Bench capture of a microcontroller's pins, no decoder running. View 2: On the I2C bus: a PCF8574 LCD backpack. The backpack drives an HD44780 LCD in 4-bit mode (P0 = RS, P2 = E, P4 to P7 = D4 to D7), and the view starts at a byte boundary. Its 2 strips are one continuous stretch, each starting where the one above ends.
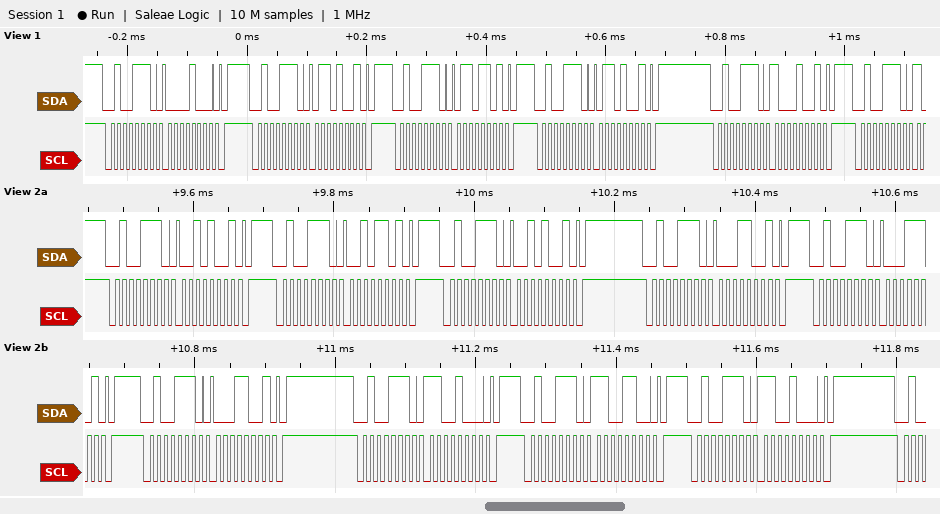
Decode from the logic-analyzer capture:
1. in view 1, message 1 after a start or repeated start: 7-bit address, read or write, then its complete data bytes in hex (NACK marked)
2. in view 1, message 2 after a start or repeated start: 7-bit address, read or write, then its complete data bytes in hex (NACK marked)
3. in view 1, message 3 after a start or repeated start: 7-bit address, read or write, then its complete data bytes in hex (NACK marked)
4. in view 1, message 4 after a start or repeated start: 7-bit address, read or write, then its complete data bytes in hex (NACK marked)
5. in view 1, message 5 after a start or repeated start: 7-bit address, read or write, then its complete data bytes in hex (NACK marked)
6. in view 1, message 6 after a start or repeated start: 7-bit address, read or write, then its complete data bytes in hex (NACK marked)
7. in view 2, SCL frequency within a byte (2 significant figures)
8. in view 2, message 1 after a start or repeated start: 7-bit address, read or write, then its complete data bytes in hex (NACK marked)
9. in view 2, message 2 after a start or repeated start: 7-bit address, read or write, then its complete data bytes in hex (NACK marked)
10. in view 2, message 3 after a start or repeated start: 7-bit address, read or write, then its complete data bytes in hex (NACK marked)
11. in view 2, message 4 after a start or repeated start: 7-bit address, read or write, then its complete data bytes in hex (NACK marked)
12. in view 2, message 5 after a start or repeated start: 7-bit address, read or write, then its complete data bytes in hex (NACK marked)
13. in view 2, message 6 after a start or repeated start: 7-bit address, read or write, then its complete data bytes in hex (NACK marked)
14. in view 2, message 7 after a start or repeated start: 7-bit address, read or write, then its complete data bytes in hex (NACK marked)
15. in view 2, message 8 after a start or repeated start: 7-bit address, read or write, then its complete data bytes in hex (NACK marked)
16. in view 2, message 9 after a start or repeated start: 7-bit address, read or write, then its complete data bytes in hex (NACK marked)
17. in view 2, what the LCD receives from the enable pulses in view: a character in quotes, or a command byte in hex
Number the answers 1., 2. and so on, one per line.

1. 0x27 write: 08
2. 0x27 write: 69
3. 0x27 write: 6D
4. 0x27 write: 69
5. 0x27 write: 89
6. 0x27 write
7. 100 kHz
8. 0x27 write: 29
9. 0x27 write: 2D
10. 0x27 write: 29
11. 0x27 write: 19
12. 0x27 write: 1D
13. 0x27 write: 19
14. 0x27 write: C8
15. 0x27 write: CC
16. 0x27 write: C8
17. '!'
